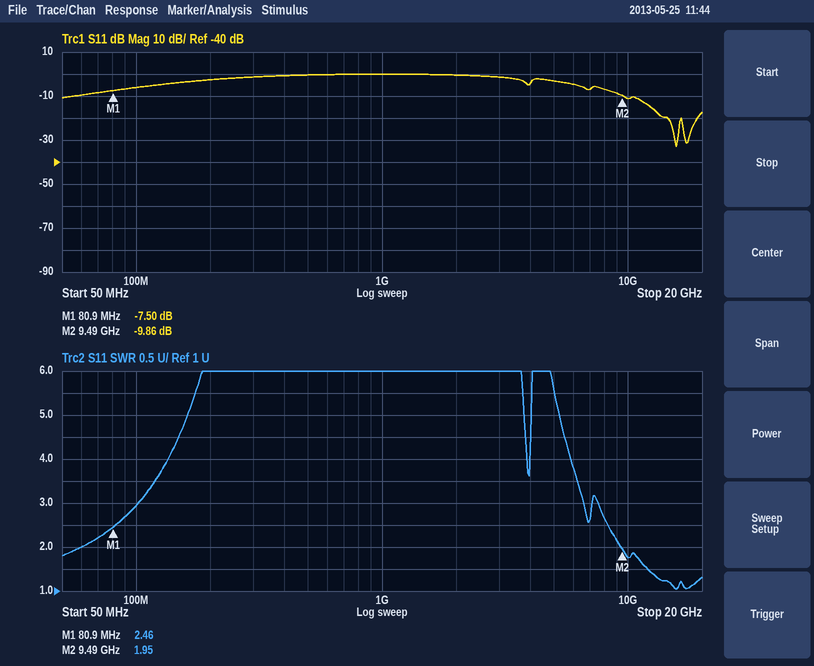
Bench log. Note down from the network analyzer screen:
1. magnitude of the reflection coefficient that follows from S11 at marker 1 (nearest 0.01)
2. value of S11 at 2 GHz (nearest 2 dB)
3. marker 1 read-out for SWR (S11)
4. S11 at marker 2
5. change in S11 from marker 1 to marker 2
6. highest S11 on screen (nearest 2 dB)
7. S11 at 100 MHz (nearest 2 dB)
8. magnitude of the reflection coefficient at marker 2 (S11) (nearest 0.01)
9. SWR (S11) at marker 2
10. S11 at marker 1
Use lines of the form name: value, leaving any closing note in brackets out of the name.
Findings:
magnitude of the reflection coefficient that follows from S11 at marker 1: 0.42
value of S11 at 2 GHz: 0 dB
marker 1 read-out for SWR: 2.46
S11 at marker 2: -9.86 dB
change in S11 from marker 1 to marker 2: -2.36 dB
highest S11 on screen: 0 dB
S11 at 100 MHz: -6 dB
magnitude of the reflection coefficient at marker 2 (S11): 0.32
SWR (S11) at marker 2: 1.95
S11 at marker 1: -7.50 dB
